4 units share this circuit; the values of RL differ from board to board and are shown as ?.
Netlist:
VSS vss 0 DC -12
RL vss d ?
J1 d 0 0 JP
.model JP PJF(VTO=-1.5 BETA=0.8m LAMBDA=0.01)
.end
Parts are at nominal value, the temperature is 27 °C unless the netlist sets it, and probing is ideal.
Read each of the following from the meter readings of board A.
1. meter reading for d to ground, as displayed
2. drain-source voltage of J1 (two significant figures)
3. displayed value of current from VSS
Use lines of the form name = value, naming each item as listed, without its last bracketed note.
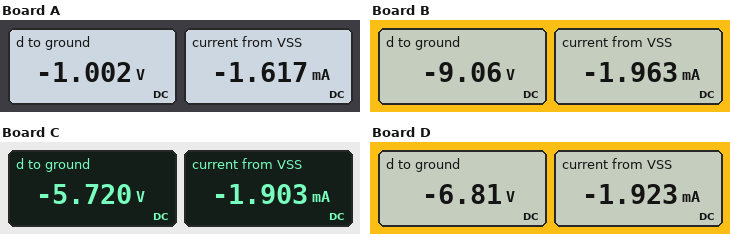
meter reading for d to ground, as displayed = -1.002 V
drain-source voltage of J1 = -1.0 V
displayed value of current from VSS = -1.617 mA
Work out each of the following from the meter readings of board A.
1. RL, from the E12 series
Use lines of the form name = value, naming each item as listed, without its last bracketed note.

RL, from the E12 series = 6.8 kΩ
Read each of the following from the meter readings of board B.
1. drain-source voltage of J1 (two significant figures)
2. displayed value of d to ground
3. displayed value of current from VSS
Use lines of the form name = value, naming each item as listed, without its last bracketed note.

drain-source voltage of J1 = -9.1 V
displayed value of d to ground = -9.06 V
displayed value of current from VSS = -1.963 mA
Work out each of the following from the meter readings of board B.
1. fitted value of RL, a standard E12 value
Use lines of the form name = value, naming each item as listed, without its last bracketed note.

fitted value of RL, a standard E12 value = 1.5 kΩ
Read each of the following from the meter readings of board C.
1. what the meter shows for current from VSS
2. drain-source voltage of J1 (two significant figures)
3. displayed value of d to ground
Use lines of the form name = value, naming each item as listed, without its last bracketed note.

what the meter shows for current from VSS = -1.903 mA
drain-source voltage of J1 = -5.7 V
displayed value of d to ground = -5.720 V
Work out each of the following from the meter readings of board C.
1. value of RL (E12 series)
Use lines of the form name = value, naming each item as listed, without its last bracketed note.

value of RL = 3.3 kΩ
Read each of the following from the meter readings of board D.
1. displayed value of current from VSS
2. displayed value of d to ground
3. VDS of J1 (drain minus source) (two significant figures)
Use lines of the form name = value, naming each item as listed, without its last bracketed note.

displayed value of current from VSS = -1.923 mA
displayed value of d to ground = -6.81 V
VDS of J1 (drain minus source) = -6.8 V
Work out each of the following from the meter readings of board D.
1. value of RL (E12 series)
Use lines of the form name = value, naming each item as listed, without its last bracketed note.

value of RL = 2.7 kΩ
